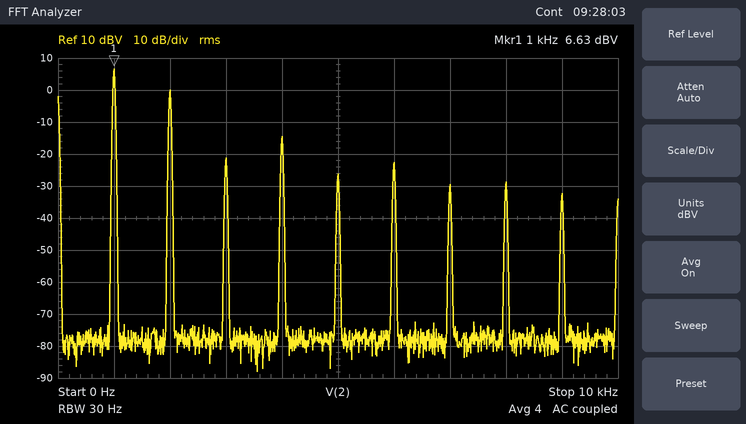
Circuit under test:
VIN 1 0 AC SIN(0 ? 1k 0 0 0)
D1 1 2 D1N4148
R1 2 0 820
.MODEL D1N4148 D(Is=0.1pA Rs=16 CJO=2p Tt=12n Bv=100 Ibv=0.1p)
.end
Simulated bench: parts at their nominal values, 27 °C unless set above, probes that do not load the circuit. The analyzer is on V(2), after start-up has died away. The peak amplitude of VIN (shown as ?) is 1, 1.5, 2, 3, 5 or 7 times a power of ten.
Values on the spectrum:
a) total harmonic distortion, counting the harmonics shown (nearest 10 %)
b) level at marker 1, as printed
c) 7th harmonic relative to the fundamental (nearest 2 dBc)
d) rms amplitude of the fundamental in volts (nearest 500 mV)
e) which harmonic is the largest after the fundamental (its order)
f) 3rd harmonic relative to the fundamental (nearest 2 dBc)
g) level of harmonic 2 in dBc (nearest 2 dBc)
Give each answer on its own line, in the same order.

50 %
6.63 dBV
-36 dBc
2.0 V
2
-28 dBc
-6 dBc
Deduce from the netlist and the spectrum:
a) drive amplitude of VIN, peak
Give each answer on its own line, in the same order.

7 V
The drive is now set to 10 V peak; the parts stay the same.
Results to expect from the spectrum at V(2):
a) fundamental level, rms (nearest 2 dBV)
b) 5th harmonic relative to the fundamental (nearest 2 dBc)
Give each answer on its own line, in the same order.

10 dBV
-36 dBc
